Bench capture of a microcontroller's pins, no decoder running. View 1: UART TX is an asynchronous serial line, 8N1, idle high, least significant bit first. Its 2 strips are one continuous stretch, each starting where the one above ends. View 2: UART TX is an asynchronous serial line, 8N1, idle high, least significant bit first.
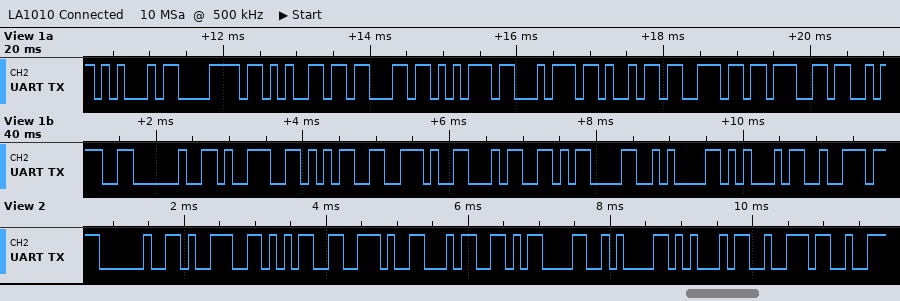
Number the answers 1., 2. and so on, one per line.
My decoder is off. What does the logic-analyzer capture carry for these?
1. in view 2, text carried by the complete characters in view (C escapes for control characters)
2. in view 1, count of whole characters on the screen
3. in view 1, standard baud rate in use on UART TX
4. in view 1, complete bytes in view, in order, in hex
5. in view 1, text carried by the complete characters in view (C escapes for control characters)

1. " 95.4\r\nEr"
2. 19
3. 9600 baud
4. 45 78 65 63 75 74 69 6E 67 3A 20 39 35 2E 34 0D 0A 45 72
5. "Executing: 95.4\r\nEr"
